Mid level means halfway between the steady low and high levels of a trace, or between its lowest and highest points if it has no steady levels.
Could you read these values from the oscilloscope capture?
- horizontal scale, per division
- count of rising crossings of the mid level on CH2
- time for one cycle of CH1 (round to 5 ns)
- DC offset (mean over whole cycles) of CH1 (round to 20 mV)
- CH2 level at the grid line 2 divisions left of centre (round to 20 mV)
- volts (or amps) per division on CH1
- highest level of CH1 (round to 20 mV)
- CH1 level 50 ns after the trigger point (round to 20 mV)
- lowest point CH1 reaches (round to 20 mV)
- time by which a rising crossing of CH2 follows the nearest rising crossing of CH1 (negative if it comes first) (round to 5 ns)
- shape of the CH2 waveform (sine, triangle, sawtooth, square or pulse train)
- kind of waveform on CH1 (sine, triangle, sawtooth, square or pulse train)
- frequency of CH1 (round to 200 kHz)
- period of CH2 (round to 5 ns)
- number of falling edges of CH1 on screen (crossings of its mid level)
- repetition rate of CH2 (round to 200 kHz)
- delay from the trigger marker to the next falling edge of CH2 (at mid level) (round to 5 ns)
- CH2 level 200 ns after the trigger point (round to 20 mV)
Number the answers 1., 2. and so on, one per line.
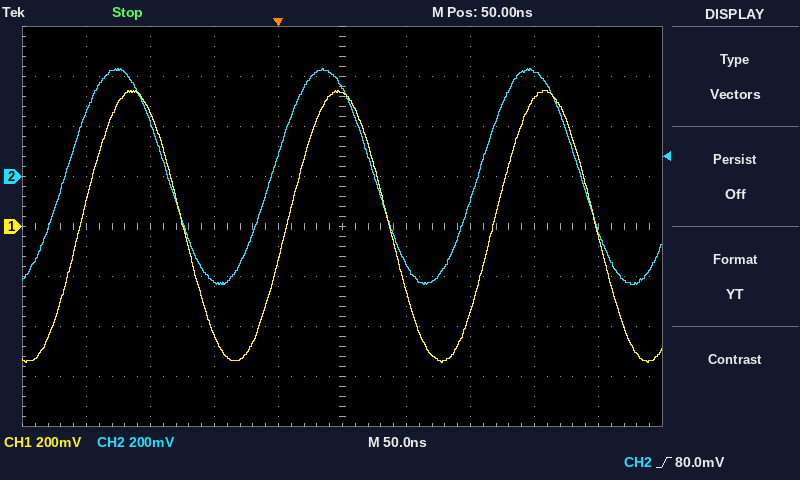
1. 50 ns
2. 3
3. 160 ns
4. 0 mV
5. -420 mV
6. 200 mV
7. 540 mV
8. 540 mV
9. -540 mV
10. -10 ns
11. sine
12. sine
13. 6.2 MHz
14. 160 ns
15. 3
16. 6.2 MHz
17. 75 ns
18. 420 mV
